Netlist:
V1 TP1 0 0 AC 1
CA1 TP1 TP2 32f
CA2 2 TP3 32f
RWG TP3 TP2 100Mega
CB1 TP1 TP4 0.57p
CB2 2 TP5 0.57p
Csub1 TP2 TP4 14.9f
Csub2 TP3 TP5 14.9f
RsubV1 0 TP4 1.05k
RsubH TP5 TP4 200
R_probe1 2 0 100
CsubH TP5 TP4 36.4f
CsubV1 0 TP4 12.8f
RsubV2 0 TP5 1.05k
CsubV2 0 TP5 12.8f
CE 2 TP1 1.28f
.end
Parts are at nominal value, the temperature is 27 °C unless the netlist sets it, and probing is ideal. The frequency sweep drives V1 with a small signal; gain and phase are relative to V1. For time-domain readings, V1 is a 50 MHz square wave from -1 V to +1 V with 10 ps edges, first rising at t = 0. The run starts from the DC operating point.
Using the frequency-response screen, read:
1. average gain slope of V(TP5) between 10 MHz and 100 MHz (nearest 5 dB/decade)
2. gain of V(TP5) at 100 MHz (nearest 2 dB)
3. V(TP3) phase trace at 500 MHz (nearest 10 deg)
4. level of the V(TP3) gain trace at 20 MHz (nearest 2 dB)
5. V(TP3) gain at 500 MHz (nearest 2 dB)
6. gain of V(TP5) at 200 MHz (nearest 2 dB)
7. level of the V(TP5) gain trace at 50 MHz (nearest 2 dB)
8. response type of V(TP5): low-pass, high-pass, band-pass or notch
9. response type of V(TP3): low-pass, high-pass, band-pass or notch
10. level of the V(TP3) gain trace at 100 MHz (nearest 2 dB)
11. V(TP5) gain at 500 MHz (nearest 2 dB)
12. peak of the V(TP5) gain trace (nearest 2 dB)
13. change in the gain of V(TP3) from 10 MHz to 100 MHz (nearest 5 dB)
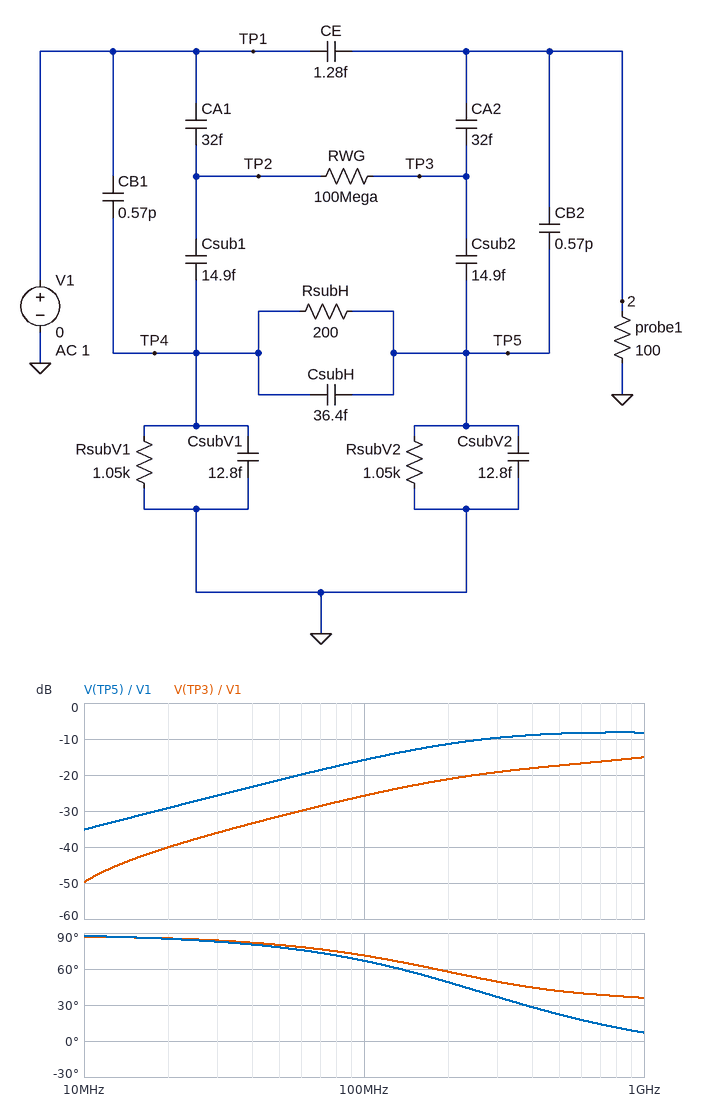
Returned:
20 dB/decade
-16 dB
40 deg
-40 dB
-18 dB
-12 dB
-22 dB
high-pass
high-pass
-26 dB
-8 dB
-8 dB
25 dB
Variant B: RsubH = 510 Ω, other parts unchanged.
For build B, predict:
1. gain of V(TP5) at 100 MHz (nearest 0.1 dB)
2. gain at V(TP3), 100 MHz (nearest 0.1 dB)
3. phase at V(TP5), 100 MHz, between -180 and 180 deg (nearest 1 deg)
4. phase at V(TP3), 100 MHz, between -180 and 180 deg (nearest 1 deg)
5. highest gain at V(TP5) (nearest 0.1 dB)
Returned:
-17.0 dB
-26.9 dB
65 deg
69 deg
-10.3 dB
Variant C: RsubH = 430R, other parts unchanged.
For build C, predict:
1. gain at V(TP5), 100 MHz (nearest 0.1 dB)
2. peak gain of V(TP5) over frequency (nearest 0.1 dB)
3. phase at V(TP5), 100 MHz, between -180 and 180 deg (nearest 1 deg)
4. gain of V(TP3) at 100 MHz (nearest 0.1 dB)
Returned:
-16.7 dB
-9.8 dB
65 deg
-26.6 dB
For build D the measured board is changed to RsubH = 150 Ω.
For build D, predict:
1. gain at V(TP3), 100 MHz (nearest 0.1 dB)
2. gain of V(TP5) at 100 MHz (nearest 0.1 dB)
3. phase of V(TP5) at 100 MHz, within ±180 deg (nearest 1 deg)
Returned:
-25.6 dB
-15.6 dB
67 deg
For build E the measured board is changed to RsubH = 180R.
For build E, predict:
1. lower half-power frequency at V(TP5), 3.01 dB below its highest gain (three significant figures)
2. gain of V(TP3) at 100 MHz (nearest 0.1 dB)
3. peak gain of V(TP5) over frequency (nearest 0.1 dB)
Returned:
212 MHz
-25.7 dB
-8.0 dB
